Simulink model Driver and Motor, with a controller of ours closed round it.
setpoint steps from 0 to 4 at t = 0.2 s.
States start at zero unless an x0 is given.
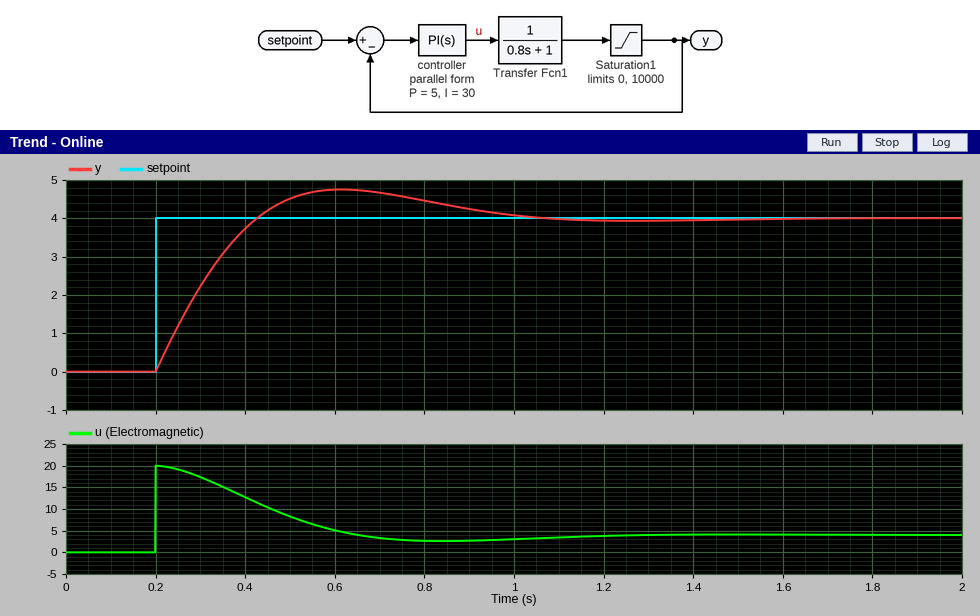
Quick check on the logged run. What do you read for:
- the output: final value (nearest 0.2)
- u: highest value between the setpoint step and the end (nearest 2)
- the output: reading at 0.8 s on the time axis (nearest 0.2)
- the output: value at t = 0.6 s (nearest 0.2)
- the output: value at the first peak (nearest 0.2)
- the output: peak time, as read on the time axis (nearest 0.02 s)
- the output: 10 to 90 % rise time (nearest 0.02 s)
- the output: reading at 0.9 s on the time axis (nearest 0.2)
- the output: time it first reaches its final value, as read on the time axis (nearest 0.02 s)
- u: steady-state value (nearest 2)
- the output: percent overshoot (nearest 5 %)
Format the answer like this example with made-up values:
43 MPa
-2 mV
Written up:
4.0
20
4.4
4.8
4.8
0.62 s
0.18 s
4.2
0.42 s
4
20 %
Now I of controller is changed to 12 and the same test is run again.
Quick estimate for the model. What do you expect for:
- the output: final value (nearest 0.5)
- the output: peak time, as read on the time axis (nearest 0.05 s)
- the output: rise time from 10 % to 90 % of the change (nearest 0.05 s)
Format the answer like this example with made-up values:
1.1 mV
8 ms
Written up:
4.0
0.85 s
0.25 s
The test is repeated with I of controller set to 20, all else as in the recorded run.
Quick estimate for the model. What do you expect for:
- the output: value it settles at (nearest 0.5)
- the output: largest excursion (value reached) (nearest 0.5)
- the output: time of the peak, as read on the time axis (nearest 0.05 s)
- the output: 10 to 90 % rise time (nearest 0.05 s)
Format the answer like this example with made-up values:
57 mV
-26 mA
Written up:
4.0
4.5
0.70 s
0.20 s
